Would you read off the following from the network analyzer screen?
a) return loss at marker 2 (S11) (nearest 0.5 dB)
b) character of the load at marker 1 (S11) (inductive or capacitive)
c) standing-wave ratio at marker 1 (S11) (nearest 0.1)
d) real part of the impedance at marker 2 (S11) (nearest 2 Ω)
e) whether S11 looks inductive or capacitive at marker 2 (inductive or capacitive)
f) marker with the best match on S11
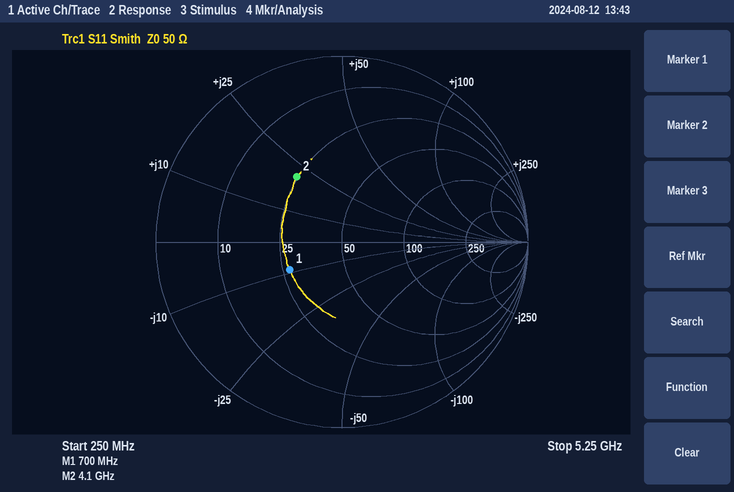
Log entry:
7.5 dB
capacitive
1.9
24 Ω
inductive
marker 1
